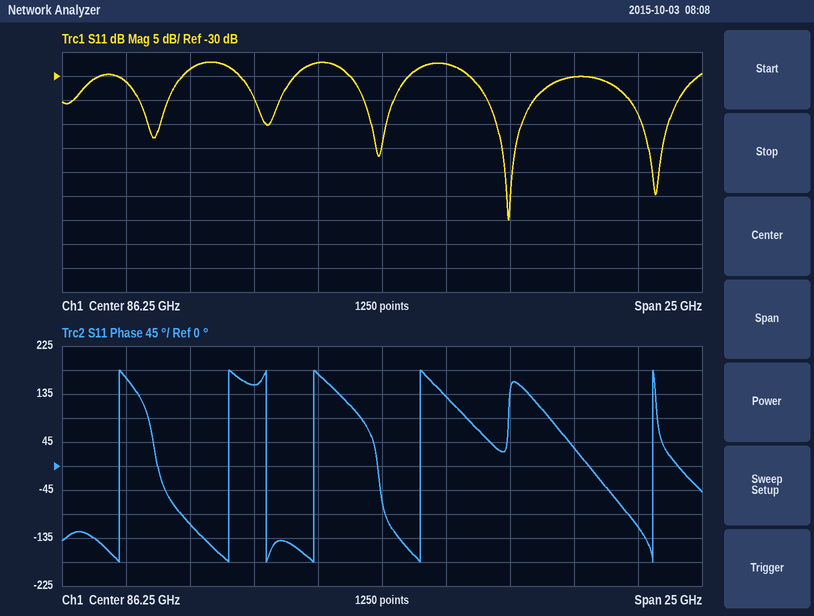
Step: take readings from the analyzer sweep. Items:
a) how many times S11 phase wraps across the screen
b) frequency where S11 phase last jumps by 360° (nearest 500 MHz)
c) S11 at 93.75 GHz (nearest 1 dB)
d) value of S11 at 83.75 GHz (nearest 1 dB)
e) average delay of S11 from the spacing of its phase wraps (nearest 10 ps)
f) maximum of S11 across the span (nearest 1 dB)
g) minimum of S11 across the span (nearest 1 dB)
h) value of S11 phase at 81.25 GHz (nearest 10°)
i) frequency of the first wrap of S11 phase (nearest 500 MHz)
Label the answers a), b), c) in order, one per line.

a) 6
b) 97.0 GHz
c) -30 dB
d) -27 dB
e) 240 ps
f) -27 dB
g) -60 dB
h) 150°
i) 76.0 GHz
